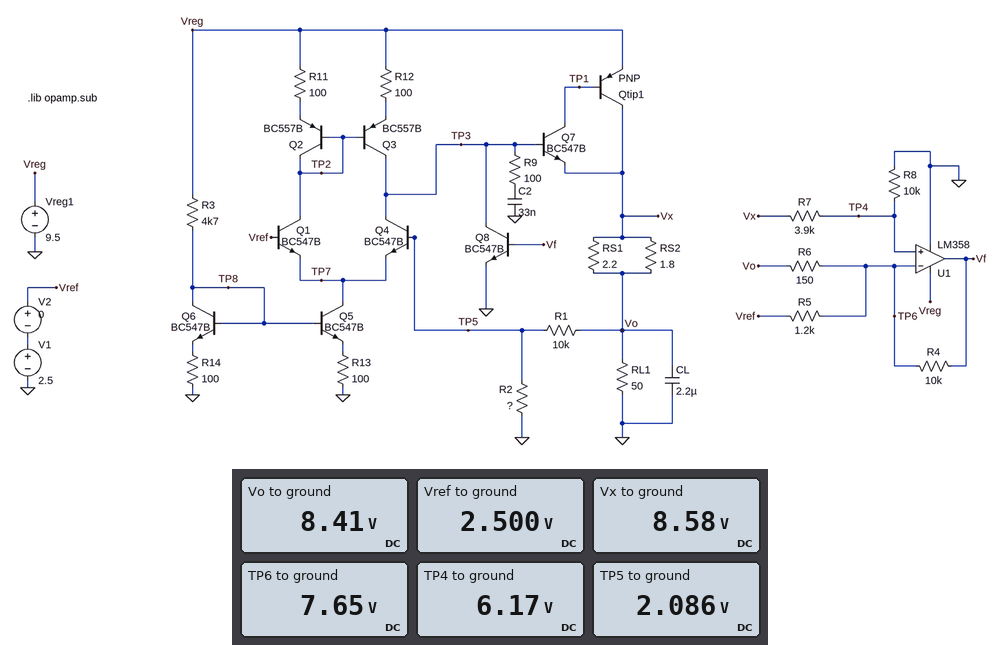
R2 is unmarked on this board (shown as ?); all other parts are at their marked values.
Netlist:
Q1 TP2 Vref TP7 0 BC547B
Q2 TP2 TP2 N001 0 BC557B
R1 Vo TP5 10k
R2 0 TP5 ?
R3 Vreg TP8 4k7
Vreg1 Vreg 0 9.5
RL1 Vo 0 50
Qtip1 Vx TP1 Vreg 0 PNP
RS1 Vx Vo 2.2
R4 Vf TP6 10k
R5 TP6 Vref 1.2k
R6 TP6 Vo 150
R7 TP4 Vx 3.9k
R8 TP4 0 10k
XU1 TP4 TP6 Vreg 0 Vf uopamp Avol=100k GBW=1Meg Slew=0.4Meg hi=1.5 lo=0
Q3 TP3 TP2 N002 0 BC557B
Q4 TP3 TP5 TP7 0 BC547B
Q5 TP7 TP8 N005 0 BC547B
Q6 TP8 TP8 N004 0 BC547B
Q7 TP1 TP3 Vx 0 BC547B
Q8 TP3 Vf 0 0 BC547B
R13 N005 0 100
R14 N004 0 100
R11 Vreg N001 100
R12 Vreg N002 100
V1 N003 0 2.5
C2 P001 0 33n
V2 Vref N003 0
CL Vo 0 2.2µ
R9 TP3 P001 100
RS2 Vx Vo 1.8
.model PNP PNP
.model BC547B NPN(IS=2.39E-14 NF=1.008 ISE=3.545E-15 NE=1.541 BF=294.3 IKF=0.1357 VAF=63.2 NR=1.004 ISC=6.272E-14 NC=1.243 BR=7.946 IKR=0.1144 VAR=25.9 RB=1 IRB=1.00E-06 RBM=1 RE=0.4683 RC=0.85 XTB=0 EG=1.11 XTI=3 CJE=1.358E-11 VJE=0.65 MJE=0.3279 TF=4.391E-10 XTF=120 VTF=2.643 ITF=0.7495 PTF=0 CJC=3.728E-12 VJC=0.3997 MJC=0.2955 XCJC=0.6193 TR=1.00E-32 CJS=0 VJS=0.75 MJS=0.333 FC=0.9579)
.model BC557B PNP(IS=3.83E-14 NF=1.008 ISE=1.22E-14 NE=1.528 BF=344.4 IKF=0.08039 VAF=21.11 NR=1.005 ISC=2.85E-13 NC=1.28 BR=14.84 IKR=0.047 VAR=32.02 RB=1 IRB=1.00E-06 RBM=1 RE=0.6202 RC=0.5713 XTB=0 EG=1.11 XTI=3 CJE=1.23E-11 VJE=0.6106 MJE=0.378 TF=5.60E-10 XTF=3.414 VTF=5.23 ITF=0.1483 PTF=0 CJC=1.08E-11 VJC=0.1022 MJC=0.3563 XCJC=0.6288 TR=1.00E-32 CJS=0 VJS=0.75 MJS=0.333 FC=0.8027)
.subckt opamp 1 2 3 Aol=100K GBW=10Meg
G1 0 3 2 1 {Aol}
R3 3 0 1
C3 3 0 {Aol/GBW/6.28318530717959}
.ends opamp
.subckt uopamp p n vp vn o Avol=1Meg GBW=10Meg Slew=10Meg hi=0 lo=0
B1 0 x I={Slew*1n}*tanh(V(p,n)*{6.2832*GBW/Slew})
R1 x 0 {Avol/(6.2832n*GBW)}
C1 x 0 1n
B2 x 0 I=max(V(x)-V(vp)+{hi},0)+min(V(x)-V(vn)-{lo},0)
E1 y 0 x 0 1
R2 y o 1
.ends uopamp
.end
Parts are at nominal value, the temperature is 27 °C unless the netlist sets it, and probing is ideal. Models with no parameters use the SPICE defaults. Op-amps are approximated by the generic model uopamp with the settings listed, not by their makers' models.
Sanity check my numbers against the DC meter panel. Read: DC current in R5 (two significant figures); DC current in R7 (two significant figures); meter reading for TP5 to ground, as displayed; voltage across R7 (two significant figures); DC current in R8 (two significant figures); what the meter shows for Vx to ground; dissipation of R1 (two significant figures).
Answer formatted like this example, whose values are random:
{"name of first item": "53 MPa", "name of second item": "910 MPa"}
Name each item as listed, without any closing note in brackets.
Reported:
{"DC current in R5": "4.3 mA", "DC current in R7": "620 µA", "meter reading for TP5 to ground, as displayed": "2.086 V", "voltage across R7": "2.4 V", "DC current in R8": "620 µA", "what the meter shows for Vx to ground": "8.58 V", "dissipation of R1": "4.0 mW"}
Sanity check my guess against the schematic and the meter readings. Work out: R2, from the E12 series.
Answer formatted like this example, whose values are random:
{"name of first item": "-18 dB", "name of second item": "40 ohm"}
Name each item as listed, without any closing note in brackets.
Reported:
{"R2, from the E12 series": "3.3 kΩ"}
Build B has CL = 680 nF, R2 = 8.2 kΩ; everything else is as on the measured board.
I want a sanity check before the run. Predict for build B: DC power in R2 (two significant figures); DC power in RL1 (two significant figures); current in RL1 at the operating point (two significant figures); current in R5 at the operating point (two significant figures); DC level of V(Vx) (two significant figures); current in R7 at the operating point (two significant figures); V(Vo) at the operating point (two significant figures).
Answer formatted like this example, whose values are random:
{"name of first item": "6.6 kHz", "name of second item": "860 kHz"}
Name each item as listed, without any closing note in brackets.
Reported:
{"DC power in R2": "760 µW", "DC power in RL1": "620 mW", "current in RL1 at the operating point": "110 mA", "current in R5 at the operating point": "2.2 mA", "DC level of V(Vx)": "5.7 V", "current in R7 at the operating point": "410 µA", "V(Vo) at the operating point": "5.6 V"}
